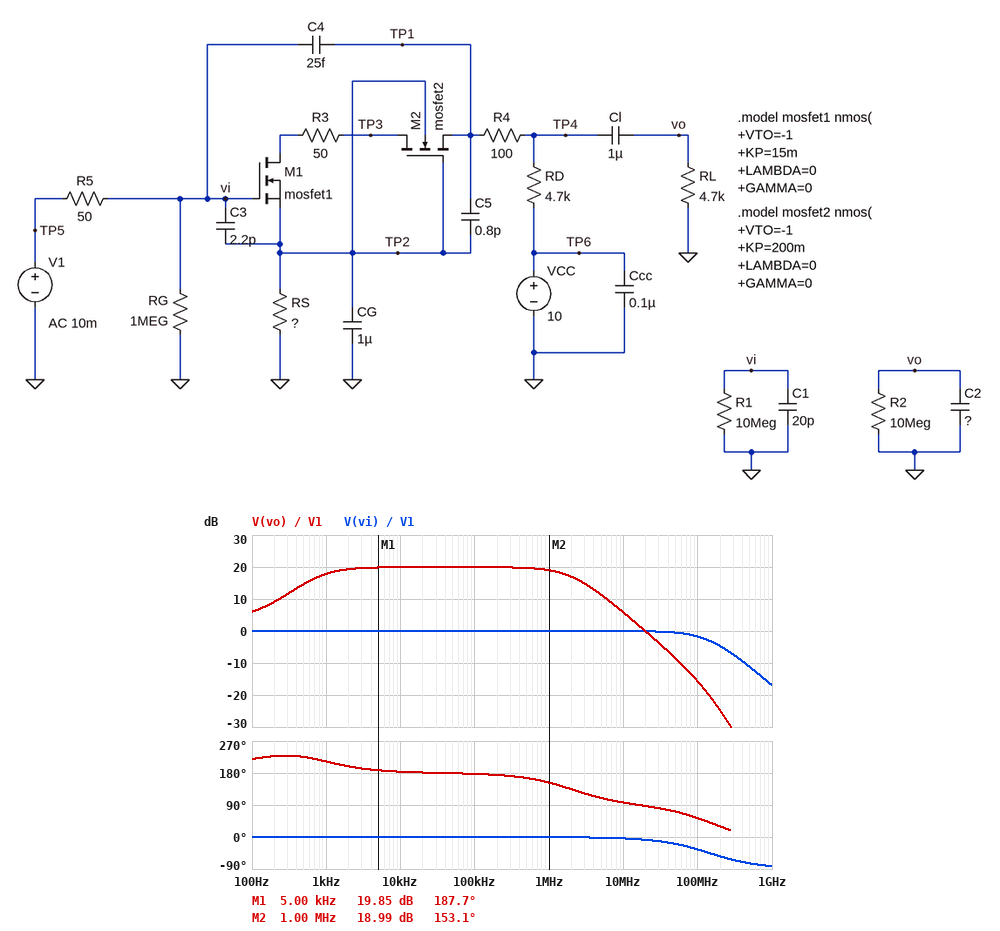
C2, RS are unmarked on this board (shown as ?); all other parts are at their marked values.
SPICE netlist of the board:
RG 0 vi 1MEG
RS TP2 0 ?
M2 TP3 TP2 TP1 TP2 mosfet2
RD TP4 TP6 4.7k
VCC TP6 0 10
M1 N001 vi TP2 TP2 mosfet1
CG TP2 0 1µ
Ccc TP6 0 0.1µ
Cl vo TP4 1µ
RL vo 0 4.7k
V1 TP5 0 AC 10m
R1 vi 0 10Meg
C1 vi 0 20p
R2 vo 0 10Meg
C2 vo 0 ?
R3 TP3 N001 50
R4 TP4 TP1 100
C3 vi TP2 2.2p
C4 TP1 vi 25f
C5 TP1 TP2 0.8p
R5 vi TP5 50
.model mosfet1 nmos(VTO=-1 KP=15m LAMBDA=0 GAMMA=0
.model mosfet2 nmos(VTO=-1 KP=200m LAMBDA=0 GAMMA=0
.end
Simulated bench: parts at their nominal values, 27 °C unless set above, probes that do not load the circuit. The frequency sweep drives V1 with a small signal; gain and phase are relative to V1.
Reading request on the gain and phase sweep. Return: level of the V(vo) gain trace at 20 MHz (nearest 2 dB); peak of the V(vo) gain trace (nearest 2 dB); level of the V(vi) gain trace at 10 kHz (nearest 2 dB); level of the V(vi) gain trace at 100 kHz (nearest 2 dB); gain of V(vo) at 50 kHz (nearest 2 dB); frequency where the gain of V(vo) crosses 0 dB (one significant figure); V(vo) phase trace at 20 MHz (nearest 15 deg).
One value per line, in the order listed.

0 dB
20 dB
0 dB
0 dB
20 dB
20 MHz
90 deg
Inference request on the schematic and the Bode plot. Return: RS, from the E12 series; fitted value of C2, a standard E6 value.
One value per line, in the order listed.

1.2 kΩ
33 pF
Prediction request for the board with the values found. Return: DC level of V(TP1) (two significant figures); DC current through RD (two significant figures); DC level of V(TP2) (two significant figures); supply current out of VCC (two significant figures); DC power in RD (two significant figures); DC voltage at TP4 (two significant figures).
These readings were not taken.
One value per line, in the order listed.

7.1 V
600 µA
720 mV
600 µA
1.7 mW
7.2 V
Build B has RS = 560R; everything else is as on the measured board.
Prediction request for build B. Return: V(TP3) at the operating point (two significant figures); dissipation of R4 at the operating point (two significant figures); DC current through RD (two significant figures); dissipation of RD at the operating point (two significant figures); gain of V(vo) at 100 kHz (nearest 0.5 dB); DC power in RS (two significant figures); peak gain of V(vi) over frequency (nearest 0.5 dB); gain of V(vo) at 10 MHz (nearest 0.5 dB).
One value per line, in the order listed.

1.5 V
120 µW
1.1 mA
5.7 mW
22.5 dB
680 µW
0 dB
8.5 dB
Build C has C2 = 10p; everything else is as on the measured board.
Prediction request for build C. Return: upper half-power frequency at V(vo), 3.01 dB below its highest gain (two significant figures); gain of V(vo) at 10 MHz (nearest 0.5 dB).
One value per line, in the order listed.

6.2 MHz
14.5 dB
